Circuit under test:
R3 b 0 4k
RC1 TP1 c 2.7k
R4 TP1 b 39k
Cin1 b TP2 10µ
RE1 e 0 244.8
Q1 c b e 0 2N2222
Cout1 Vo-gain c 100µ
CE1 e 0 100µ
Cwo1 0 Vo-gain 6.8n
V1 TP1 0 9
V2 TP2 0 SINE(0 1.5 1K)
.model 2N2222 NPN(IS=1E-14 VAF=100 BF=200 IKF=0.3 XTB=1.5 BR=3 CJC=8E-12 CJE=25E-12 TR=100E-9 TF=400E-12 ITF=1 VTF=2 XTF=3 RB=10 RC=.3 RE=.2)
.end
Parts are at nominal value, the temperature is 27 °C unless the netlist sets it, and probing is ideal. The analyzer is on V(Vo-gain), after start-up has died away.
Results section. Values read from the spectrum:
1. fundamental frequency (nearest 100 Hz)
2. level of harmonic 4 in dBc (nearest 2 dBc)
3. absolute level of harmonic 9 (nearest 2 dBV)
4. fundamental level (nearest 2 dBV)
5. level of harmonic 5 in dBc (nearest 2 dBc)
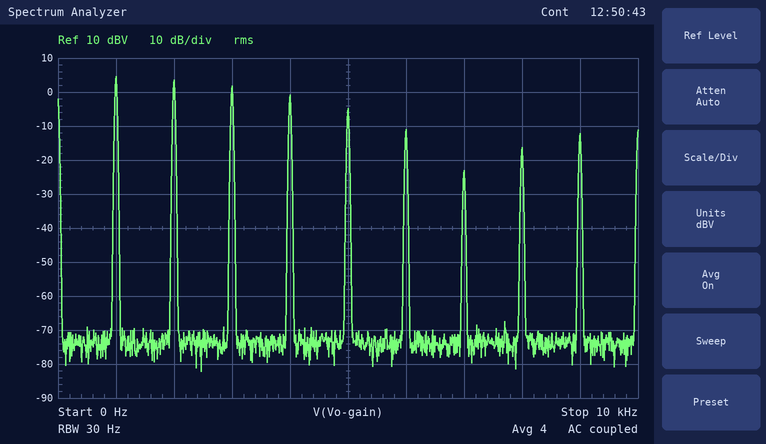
1.0 kHz
-6 dBc
-12 dBV
4 dBV
-10 dBc
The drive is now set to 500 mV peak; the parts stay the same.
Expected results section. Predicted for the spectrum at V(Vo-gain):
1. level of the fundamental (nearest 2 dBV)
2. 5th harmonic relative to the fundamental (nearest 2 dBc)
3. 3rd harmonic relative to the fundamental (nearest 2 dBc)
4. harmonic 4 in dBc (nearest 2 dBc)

6 dBV
-16 dBc
-4 dBc
-8 dBc
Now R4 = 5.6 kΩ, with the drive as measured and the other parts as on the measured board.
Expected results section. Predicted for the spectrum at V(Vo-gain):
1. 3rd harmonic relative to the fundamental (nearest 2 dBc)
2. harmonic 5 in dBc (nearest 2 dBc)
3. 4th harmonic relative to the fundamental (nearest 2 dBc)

-6 dBc
-32 dBc
-12 dBc
